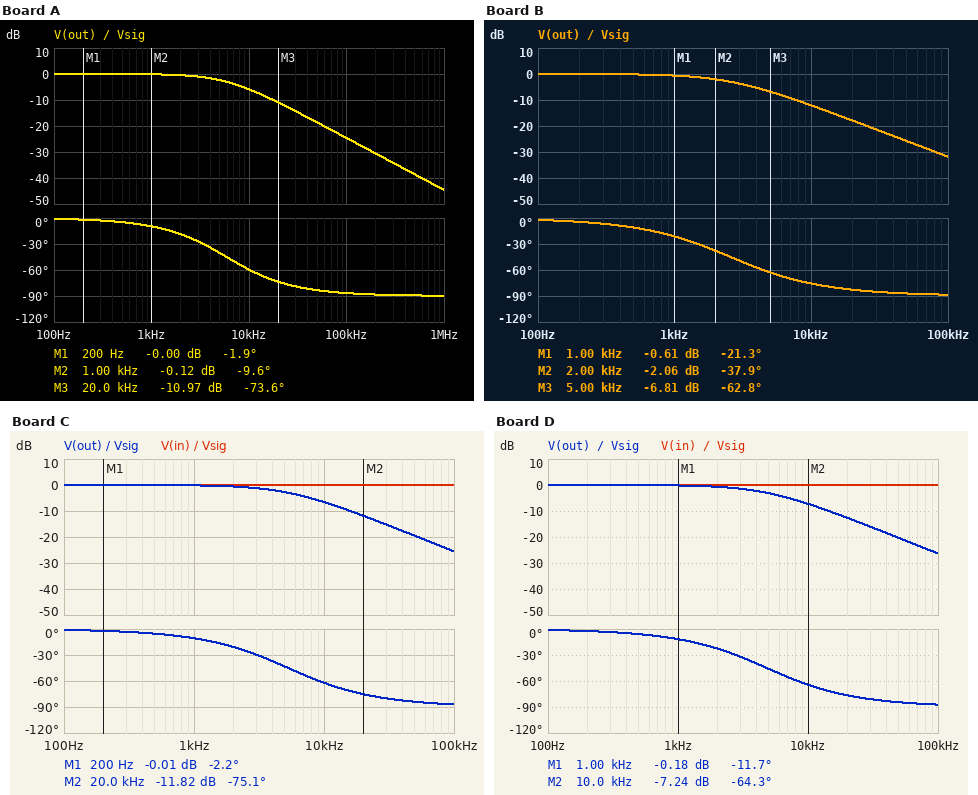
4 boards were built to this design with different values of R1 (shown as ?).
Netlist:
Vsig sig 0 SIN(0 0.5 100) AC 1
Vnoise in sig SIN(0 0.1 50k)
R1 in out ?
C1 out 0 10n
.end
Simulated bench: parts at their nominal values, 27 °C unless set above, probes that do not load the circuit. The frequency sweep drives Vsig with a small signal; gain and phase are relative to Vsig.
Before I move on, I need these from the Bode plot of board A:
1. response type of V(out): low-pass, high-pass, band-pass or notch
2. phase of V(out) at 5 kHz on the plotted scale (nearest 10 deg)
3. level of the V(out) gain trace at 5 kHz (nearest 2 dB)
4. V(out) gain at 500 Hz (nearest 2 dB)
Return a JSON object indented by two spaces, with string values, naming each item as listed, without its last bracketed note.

{
  "response type of V(out): low-pass, high-pass, band-pass or notch": "low-pass",
  "phase of V(out) at 5 kHz on the plotted scale": "-40 deg",
  "level of the V(out) gain trace at 5 kHz": "-2 dB",
  "V(out) gain at 500 Hz": "0 dB"
}
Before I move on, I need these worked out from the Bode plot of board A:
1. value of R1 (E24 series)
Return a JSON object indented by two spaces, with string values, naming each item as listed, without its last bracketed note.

{
  "value of R1": "2.7 kΩ"
}
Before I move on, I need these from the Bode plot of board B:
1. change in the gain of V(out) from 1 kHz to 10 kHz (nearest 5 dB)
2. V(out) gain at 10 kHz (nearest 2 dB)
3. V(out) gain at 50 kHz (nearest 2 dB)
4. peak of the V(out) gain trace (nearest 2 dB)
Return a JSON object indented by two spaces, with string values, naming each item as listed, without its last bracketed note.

{
  "change in the gain of V(out) from 1 kHz to 10 kHz": "-10 dB",
  "V(out) gain at 10 kHz": "-12 dB",
  "V(out) gain at 50 kHz": "-26 dB",
  "peak of the V(out) gain trace": "0 dB"
}
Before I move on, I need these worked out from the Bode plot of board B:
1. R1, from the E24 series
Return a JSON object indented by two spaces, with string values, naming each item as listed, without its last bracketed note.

{
  "R1, from the E24 series": "6.2 kΩ"
}
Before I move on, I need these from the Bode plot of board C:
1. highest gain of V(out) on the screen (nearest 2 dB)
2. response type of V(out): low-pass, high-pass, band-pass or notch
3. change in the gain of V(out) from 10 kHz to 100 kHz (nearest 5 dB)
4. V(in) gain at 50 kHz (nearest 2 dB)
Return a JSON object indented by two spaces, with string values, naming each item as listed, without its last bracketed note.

{
  "highest gain of V(out) on the screen": "0 dB",
  "response type of V(out): low-pass, high-pass, band-pass or notch": "low-pass",
  "change in the gain of V(out) from 10 kHz to 100 kHz": "-20 dB",
  "V(in) gain at 50 kHz": "0 dB"
}
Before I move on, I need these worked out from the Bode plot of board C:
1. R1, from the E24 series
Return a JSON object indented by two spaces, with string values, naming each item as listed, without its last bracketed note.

{
  "R1, from the E24 series": "3 kΩ"
}
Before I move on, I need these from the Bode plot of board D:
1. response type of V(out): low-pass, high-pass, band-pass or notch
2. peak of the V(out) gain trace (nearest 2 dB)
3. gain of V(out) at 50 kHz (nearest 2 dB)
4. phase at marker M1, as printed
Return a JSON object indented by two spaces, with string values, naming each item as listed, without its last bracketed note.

{
  "response type of V(out): low-pass, high-pass, band-pass or notch": "low-pass",
  "peak of the V(out) gain trace": "0 dB",
  "gain of V(out) at 50 kHz": "-20 dB",
  "phase at marker M1, as printed": "-11.7 deg"
}
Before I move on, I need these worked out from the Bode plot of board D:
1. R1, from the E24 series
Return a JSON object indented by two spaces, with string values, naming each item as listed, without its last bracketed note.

{
  "R1, from the E24 series": "3.3 kΩ"
}
